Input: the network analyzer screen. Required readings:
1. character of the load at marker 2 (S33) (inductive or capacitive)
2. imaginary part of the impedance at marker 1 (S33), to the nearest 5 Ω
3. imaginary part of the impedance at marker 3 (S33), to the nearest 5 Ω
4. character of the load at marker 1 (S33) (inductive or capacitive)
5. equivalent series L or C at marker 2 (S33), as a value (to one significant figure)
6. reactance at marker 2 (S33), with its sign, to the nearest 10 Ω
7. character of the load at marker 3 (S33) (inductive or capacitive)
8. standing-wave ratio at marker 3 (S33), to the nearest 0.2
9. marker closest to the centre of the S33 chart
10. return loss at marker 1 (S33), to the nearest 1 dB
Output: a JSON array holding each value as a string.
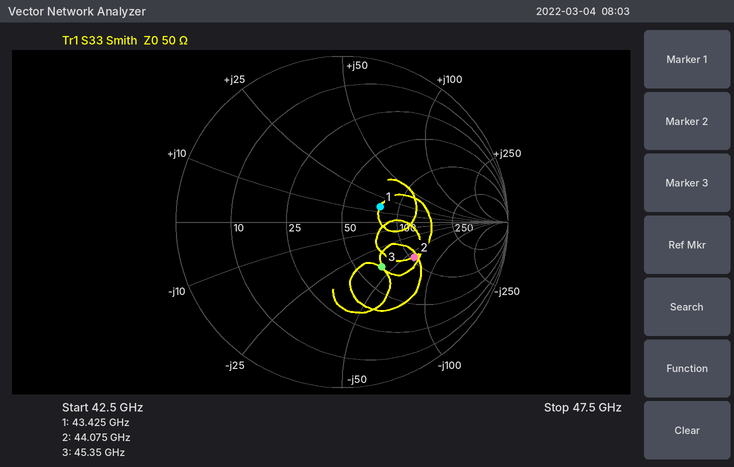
["capacitive", "+15 Ω", "-40 Ω", "inductive", "60 fF", "-60 Ω", "capacitive", "2.2", "marker 1", "12 dB"]
